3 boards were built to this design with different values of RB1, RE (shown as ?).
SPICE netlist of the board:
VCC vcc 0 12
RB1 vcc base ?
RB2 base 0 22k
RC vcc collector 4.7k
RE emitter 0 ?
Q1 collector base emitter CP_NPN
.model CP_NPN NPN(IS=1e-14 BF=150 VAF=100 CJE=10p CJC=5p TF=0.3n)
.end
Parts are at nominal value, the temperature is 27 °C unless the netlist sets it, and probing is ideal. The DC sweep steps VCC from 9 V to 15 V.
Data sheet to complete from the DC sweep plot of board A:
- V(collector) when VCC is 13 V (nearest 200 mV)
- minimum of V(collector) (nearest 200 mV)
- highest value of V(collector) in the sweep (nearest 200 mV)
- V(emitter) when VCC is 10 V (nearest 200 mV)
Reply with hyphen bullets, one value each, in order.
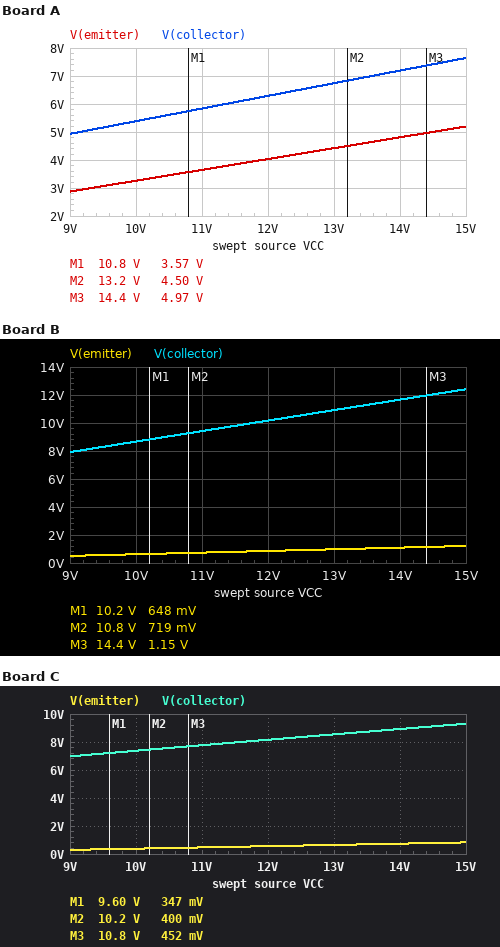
- 6.8 V
- 5.0 V
- 7.6 V
- 3.2 V
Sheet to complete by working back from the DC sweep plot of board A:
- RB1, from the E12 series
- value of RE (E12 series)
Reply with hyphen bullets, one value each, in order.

- 33 kΩ
- 3.3 kΩ
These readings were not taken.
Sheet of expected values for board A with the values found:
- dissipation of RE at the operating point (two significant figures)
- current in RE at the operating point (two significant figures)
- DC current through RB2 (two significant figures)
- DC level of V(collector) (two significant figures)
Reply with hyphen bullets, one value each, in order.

- 4.9 mW
- 1.2 mA
- 210 µA
- 6.3 V
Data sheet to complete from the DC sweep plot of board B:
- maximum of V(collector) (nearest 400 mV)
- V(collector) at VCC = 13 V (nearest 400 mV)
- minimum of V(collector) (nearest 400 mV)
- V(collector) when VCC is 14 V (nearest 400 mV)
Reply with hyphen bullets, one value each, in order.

- 12.4 V
- 10.8 V
- 8.0 V
- 11.6 V
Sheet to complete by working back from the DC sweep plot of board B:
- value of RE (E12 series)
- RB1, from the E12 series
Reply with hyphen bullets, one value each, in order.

- 2.2 kΩ
- 150 kΩ
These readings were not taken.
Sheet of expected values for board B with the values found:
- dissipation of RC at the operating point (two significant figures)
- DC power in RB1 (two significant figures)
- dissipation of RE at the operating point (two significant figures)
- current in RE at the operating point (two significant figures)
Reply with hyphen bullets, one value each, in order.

- 710 µW
- 740 µW
- 340 µW
- 390 µA
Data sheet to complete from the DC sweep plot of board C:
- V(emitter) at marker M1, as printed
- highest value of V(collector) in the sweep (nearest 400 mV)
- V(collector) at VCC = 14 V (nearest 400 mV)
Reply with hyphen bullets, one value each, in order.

- 347 mV
- 9.2 V
- 8.8 V
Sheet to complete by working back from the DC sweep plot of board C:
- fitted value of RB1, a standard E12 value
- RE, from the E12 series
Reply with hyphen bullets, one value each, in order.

- 180 kΩ
- 680 Ω
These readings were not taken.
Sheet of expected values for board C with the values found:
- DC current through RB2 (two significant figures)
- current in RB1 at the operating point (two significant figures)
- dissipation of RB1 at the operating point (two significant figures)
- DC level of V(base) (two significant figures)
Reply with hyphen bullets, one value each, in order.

- 55 µA
- 60 µA
- 650 µW
- 1.2 V
